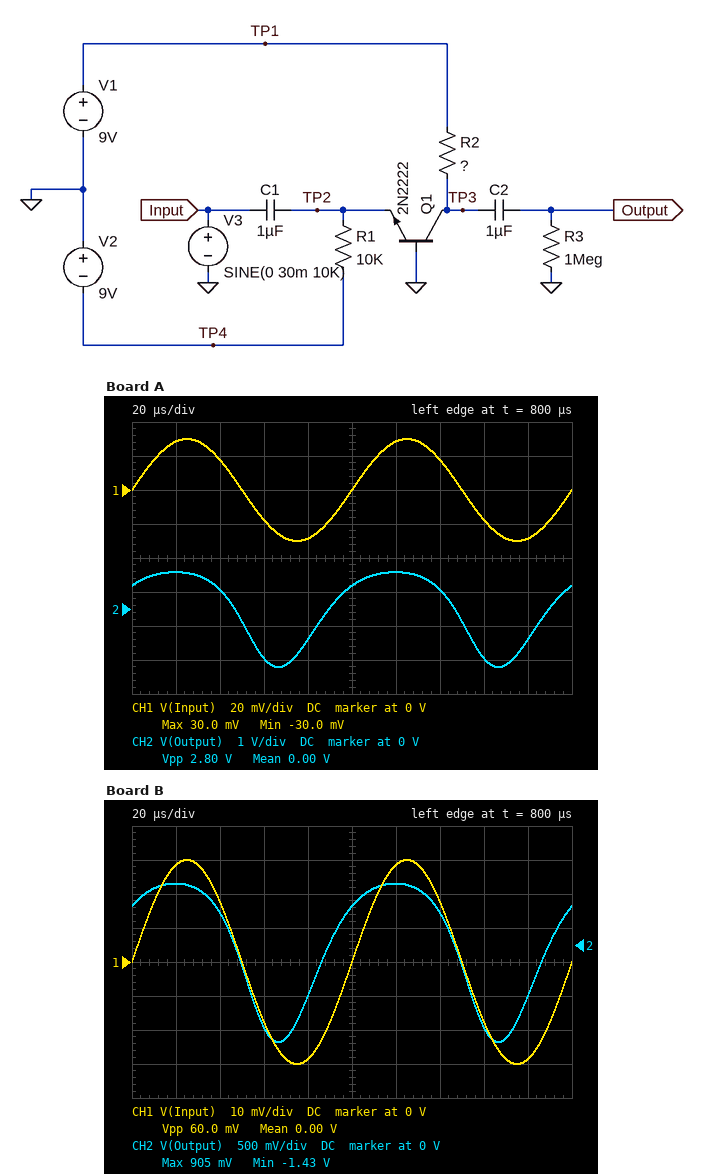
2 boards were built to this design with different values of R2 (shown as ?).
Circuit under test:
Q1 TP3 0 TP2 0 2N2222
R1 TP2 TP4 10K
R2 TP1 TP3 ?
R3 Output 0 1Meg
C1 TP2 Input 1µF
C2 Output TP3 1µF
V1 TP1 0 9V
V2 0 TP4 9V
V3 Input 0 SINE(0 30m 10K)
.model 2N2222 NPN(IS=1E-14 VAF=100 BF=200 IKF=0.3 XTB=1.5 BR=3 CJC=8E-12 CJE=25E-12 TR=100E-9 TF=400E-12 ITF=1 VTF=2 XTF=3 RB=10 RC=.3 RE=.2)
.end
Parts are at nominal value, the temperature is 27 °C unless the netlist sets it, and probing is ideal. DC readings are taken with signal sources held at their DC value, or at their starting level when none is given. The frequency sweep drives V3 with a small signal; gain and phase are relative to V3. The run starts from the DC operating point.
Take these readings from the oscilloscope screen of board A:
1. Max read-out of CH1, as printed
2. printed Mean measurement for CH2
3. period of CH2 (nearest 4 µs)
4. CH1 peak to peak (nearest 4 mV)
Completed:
30.0 mV
0.00 V
100 µs
60 mV
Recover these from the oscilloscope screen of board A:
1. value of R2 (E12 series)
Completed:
1.8 kΩ
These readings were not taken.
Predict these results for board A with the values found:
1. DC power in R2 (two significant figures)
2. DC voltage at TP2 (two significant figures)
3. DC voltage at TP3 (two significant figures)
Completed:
1.2 mW
-650 mV
7.5 V
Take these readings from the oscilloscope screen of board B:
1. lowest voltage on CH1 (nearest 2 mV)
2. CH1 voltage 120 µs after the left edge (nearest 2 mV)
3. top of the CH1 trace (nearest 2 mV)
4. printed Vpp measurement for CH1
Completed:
-30 mV
28 mV
30 mV
60.0 mV
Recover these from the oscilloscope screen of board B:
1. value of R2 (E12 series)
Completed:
1.5 kΩ
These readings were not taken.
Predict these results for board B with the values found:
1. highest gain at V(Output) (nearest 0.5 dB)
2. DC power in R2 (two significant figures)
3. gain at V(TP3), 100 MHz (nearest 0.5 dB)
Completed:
33.5 dB
1.0 mW
19.5 dB
